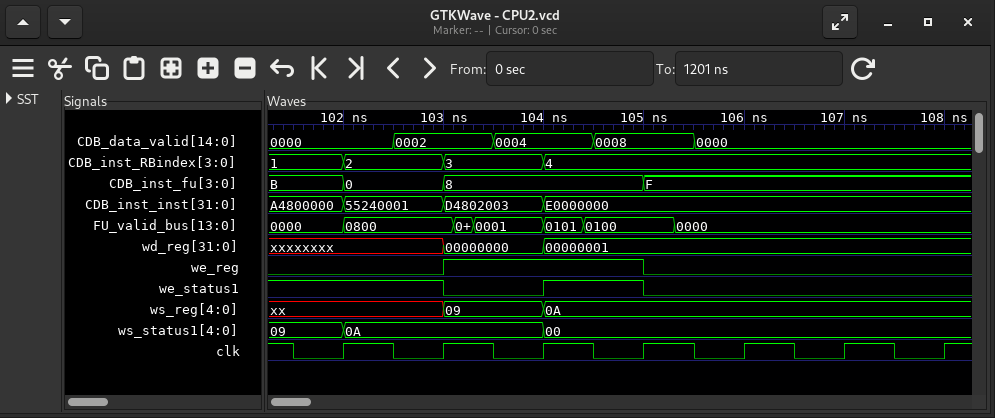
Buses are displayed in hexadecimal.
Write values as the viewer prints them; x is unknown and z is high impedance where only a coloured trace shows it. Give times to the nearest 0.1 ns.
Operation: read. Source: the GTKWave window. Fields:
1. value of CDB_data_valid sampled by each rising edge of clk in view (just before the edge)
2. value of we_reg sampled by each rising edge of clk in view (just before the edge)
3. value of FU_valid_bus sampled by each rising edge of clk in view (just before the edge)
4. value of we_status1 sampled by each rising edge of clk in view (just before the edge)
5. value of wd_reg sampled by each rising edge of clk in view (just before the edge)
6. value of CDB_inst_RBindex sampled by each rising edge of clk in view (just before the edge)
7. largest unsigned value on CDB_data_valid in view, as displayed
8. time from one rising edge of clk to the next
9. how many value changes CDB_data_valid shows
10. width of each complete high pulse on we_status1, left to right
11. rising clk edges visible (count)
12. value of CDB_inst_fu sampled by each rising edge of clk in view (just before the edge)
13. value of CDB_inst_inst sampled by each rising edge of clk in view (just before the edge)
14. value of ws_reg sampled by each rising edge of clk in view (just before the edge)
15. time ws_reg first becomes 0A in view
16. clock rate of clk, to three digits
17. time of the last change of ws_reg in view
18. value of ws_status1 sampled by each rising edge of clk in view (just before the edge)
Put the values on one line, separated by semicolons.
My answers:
0000, 0002, 0004, 0008, 0000, 0000, 0000; 0 0 1 1 0 0 0; 0000, 0800, 0001, 0100, 0000, 0000, 0000; 1 1 0 1 0 0 0; xxxxxxxx, xxxxxxxx, 00000000, 00000001, 00000001, 00000001, 00000001; 1, 2, 3, 4, 4, 4, 4; 0008; 1 ns; 4; 1 ns; 7; B, 0, 8, 8, F, F, F; A4800000, 55240001, D4802003, E0000000, E0000000, E0000000, E0000000; xx, xx, 09, 0A, 0A, 0A, 0A; 104 ns; 1.00 GHz; 104 ns; 09, 0A, 0A, 00, 00, 00, 00
